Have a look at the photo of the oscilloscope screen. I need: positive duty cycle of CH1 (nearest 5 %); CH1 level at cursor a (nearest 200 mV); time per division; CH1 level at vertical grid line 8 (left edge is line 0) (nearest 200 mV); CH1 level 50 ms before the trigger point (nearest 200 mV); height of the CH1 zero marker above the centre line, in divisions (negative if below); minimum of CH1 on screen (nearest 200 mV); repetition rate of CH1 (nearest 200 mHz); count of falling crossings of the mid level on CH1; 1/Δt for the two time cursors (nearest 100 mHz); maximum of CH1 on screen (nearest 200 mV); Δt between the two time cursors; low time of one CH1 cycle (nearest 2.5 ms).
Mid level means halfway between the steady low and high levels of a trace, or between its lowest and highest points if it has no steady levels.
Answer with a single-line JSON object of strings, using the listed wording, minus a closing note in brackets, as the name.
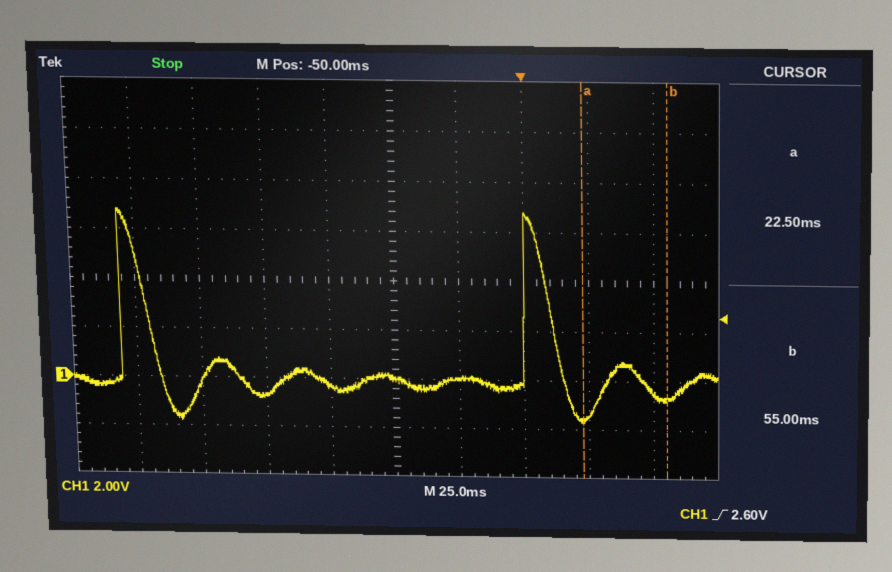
{"positive duty cycle of CH1": "5 %", "CH1 level at cursor a": "-1.6 V", "time per division": "25 ms", "CH1 level at vertical grid line 8 (left edge is line 0)": "-1.4 V", "CH1 level 50 ms before the trigger point": "0.0 V", "height of the CH1 zero marker above the centre line, in divisions": "-2.0 div", "minimum of CH1 on screen": "-1.8 V", "repetition rate of CH1": "6.4 Hz", "count of falling crossings of the mid level on CH1": "2", "1/Δt for the two time cursors": "30.8 Hz", "maximum of CH1 on screen": "6.8 V", "Δt between the two time cursors": "32.5 ms", "low time of one CH1 cycle": "145.0 ms"}
